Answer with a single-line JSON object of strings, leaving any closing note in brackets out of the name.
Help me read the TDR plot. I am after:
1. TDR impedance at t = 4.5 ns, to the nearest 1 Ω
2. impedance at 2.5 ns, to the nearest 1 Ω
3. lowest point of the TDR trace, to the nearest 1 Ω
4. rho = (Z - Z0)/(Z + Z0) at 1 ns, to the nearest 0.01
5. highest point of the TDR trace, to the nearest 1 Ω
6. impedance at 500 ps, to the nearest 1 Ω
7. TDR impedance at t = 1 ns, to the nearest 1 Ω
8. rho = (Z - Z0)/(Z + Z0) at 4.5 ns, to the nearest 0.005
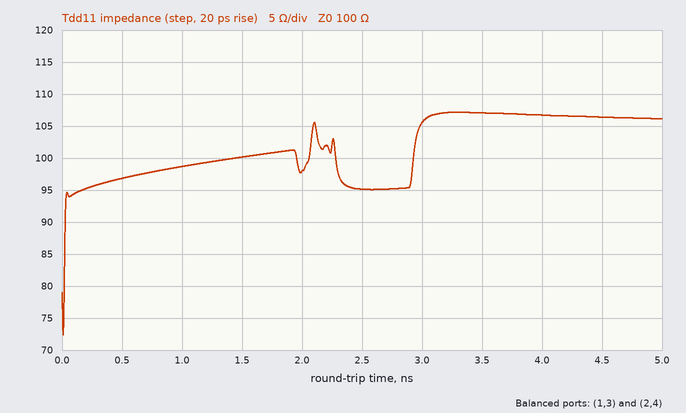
{"TDR impedance at t = 4.5 ns, to the nearest 1 Ω": "106 Ω", "impedance at 2.5 ns, to the nearest 1 Ω": "95 Ω", "lowest point of the TDR trace, to the nearest 1 Ω": "72 Ω", "rho = (Z - Z0)/(Z + Z0) at 1 ns, to the nearest 0.01": "-0.01", "highest point of the TDR trace, to the nearest 1 Ω": "107 Ω", "impedance at 500 ps, to the nearest 1 Ω": "97 Ω", "TDR impedance at t = 1 ns, to the nearest 1 Ω": "99 Ω", "rho = (Z - Z0)/(Z + Z0) at 4.5 ns, to the nearest 0.005": "+0.030"}
